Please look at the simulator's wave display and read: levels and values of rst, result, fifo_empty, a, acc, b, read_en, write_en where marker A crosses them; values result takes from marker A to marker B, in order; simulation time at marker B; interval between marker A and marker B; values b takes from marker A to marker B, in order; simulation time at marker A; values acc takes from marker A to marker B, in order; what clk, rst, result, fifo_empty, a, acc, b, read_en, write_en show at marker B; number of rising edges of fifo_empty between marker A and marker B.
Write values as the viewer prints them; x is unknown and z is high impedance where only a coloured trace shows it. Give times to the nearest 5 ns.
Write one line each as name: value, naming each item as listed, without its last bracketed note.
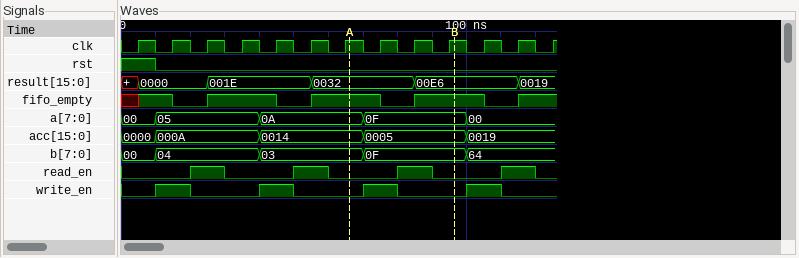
levels and values of rst, result, fifo_empty, a, acc, b, read_en, write_en where marker A crosses them: rst=0, result=0032, fifo_empty=1, a=0A, acc=0014, b=03, read_en=0, write_en=0
values result takes from marker A to marker B, in order: 0032, 00E6
simulation time at marker B: 95 ns
interval between marker A and marker B: 30 ns
values b takes from marker A to marker B, in order: 03, 0F
simulation time at marker A: 65 ns
values acc takes from marker A to marker B, in order: 0014, 0005
what clk, rst, result, fifo_empty, a, acc, b, read_en, write_en show at marker B: clk=1, rst=0, result=00E6, fifo_empty=1, a=0F, acc=0005, b=0F, read_en=0, write_en=0
number of rising edges of fifo_empty between marker A and marker B: 1
